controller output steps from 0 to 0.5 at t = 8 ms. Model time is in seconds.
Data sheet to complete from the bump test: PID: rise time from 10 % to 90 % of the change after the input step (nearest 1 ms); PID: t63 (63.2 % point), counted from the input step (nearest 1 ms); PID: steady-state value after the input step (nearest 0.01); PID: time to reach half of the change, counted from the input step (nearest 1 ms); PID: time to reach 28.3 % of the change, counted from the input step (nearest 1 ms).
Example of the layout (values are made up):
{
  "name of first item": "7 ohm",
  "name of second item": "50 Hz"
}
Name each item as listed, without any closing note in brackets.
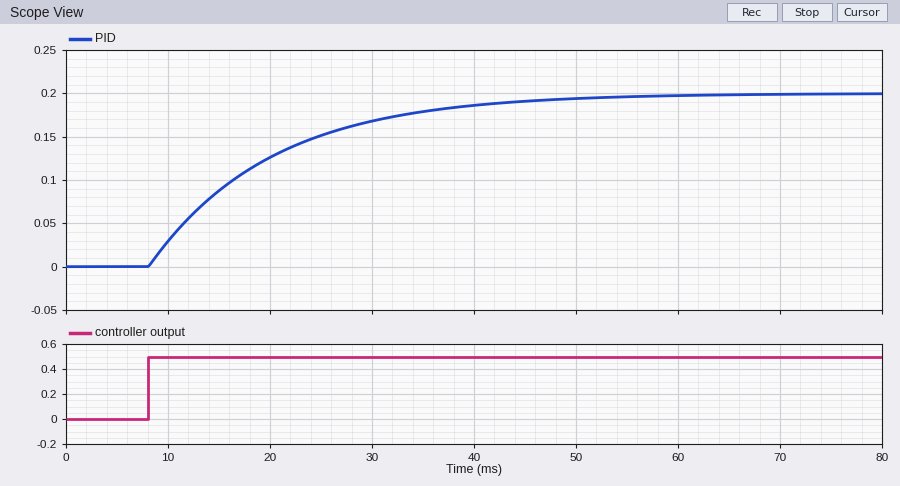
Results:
{
  "PID: rise time from 10 % to 90 % of the change after the input step": "26 ms",
  "PID: t63 (63.2 % point), counted from the input step": "12 ms",
  "PID: steady-state value after the input step": "0.20",
  "PID: time to reach half of the change, counted from the input step": "8 ms",
  "PID: time to reach 28.3 % of the change, counted from the input step": "4 ms"
}
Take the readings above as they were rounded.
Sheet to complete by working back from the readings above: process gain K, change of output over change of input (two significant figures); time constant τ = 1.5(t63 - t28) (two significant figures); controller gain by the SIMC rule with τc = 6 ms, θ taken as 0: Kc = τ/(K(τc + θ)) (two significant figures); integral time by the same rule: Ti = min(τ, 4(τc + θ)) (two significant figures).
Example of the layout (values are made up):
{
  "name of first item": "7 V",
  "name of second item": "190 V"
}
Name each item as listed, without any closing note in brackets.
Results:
{
  "process gain K, change of output over change of input": "0.40",
  "time constant τ = 1.5(t63 - t28)": "12 ms",
  "controller gain by the SIMC rule with τc = 6 ms, θ taken as 0: Kc = τ/(K(τc + θ))": "5.0",
  "integral time by the same rule: Ti = min(τ, 4(τc + θ))": "12 ms"
}
